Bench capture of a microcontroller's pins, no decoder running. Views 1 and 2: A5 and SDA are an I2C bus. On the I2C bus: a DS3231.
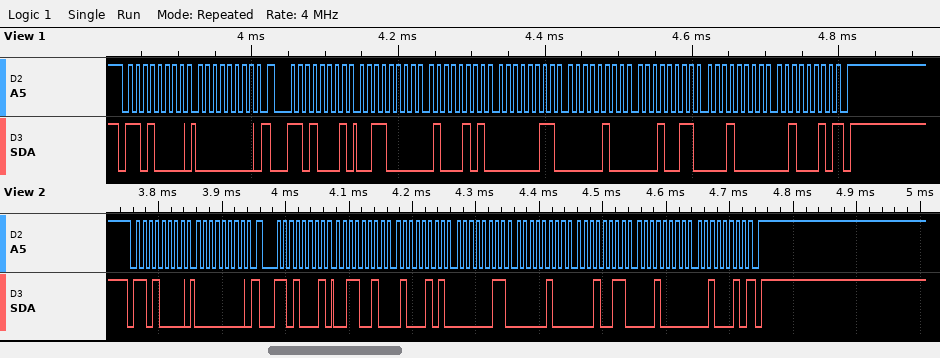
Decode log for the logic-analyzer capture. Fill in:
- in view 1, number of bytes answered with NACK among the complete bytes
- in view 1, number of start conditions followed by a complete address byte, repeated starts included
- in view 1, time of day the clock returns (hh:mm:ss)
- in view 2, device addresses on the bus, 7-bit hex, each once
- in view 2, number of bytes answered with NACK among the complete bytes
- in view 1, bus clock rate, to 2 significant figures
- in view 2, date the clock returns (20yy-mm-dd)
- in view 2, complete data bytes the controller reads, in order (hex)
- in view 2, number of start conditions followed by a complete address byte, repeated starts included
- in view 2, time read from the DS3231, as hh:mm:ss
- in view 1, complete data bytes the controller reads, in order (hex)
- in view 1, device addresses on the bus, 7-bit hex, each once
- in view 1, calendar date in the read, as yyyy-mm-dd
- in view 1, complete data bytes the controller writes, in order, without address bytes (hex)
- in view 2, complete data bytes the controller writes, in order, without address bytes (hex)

1
2
03:45:30
0x68
1
100 kHz
2022-10-13
32 45 03 04 13 10 22
2
03:45:32
30 45 03 04 13 10 22
0x68
2022-10-13
00
00
